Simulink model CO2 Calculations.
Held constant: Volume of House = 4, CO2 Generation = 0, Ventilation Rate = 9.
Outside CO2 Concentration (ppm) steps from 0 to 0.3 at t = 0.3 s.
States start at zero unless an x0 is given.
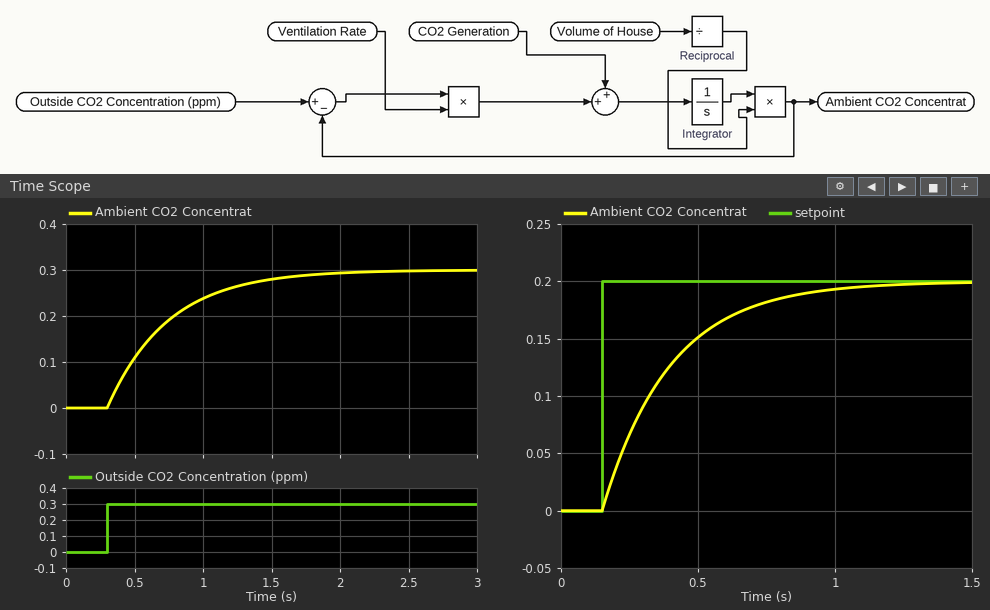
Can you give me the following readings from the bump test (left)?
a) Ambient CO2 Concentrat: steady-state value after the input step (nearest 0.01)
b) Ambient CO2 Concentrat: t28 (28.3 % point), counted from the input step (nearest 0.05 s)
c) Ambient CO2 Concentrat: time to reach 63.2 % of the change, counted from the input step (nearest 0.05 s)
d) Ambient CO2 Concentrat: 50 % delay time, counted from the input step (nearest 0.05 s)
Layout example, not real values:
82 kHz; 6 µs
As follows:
0.30; 0.15 s; 0.45 s; 0.30 s
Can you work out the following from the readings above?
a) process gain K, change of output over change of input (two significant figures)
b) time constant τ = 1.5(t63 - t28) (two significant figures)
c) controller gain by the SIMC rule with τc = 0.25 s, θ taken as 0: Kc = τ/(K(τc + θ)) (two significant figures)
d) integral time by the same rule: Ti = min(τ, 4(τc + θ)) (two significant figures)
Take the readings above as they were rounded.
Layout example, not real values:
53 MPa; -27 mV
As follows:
1.0; 0.45 s; 1.8; 0.45 s
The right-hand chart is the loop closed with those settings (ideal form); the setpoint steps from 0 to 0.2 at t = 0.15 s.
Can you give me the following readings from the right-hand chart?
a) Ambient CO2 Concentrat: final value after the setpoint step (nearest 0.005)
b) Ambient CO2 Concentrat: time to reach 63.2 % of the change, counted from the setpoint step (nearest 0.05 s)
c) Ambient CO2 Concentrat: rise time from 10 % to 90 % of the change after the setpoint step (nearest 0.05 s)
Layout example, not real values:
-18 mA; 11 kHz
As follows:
0.200; 0.25 s; 0.55 s
